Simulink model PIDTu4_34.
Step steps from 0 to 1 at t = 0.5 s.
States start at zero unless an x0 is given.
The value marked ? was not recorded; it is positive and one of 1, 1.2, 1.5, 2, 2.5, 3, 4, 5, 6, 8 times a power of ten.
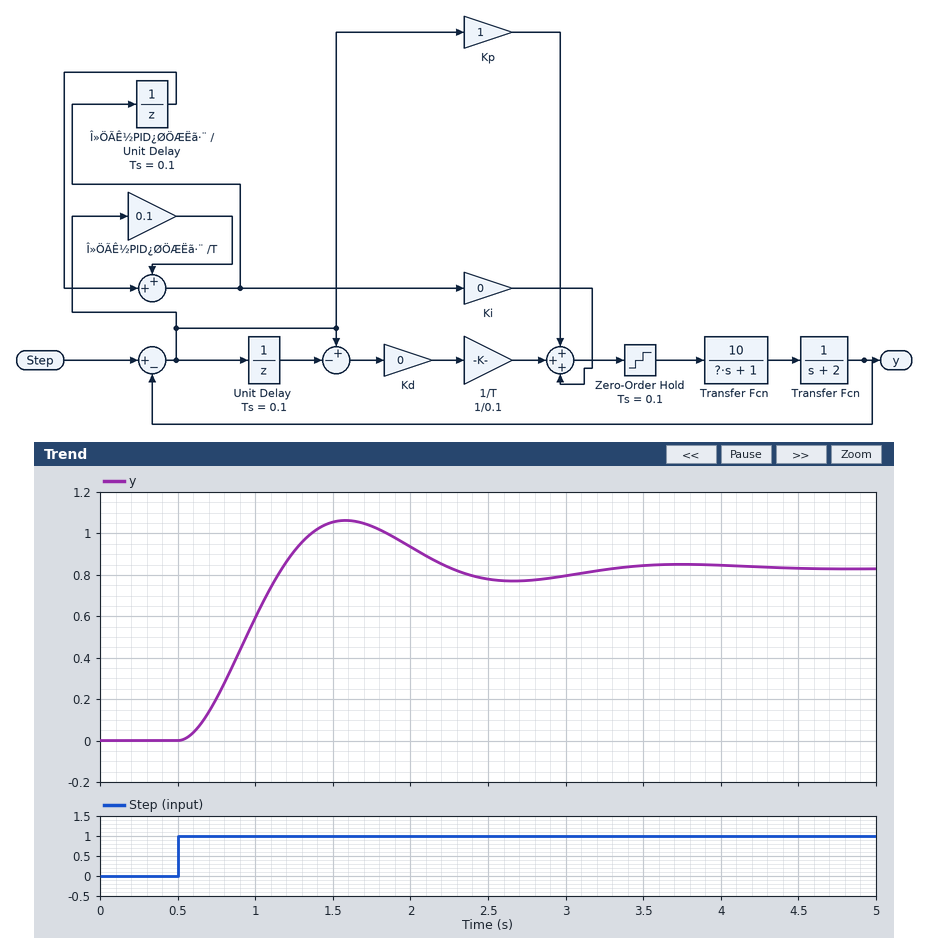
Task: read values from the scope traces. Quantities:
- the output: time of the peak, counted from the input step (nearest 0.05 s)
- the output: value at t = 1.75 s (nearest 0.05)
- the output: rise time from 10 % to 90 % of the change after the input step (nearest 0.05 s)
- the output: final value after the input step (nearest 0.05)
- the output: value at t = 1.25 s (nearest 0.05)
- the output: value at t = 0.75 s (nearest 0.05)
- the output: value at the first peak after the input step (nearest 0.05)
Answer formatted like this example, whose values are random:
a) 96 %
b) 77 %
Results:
a) 1.10 s
b) 1.05
c) 0.45 s
d) 0.85
e) 0.90
f) 0.20
g) 1.05
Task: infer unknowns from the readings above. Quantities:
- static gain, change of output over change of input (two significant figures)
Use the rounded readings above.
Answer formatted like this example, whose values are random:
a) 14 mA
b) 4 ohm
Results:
a) 0.85
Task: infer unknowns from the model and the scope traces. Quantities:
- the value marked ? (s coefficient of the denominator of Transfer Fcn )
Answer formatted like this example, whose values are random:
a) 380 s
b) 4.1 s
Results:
a) 1.2
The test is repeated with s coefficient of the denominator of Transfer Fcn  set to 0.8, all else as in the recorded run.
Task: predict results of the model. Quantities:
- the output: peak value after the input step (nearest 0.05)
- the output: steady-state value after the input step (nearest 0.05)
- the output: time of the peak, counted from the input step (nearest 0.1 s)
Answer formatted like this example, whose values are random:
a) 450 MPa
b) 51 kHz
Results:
a) 1.10
b) 0.85
c) 0.9 s
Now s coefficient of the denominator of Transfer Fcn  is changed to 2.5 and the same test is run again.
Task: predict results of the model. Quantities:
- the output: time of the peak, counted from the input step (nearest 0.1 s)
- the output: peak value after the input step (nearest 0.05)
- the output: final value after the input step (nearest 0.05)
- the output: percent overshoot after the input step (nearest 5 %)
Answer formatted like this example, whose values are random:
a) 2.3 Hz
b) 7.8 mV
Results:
a) 1.7 s
b) 0.95
c) 0.85
d) 15 %
